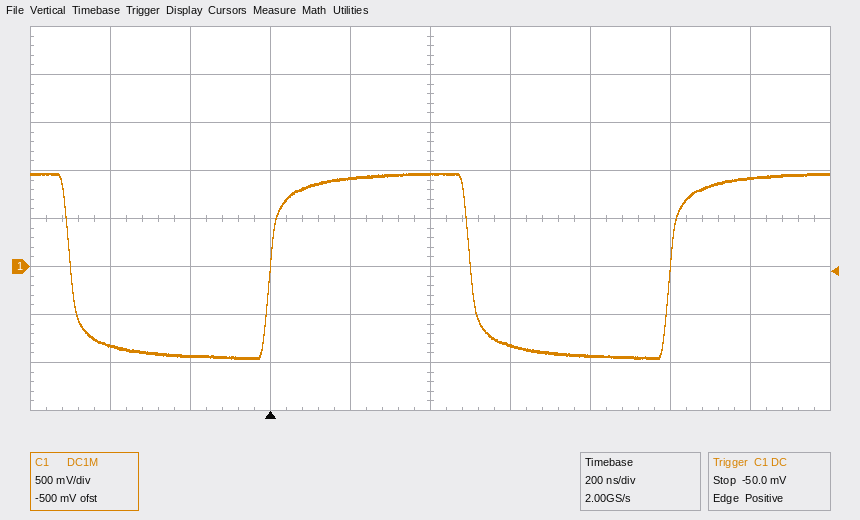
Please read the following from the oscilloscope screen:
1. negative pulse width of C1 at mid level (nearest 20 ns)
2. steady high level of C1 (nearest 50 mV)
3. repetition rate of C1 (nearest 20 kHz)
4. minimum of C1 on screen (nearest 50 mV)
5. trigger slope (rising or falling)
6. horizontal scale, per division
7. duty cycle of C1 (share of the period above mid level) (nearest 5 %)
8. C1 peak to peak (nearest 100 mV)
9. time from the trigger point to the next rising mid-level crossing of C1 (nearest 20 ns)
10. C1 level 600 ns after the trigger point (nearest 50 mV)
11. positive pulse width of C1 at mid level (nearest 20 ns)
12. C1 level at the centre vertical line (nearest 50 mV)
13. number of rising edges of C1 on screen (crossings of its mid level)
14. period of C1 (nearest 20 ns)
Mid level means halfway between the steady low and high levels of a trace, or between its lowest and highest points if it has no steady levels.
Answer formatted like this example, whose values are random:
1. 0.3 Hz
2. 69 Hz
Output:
1. 500 ns
2. 950 mV
3. 1.00 MHz
4. -950 mV
5. rising
6. 200 ns
7. 50 %
8. 1.90 V
9. 1.00 µs
10. -800 mV
11. 500 ns
12. 950 mV
13. 2
14. 1.00 µs
